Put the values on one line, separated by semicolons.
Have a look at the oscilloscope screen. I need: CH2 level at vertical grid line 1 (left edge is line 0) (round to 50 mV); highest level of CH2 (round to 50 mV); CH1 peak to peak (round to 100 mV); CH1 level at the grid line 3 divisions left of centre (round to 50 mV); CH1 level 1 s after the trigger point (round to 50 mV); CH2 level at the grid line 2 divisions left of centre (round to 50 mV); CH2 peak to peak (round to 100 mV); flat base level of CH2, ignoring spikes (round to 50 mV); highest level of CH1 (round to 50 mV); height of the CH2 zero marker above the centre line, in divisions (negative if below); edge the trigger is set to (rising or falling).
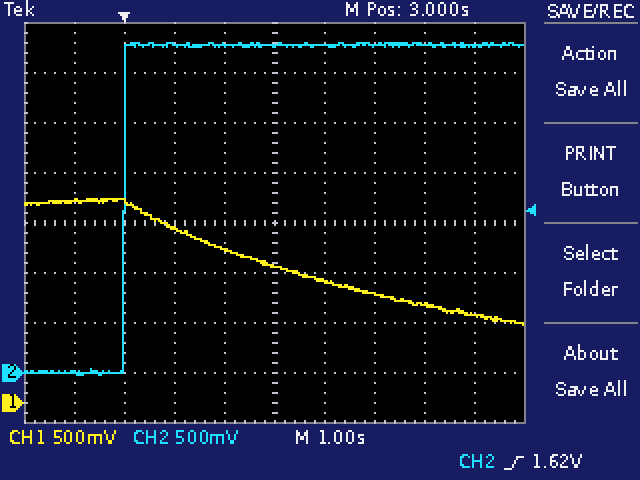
0 mV; 3.30 V; 1.30 V; 2.00 V; 1.75 V; 3.30 V; 3.30 V; 0 mV; 2.05 V; -3.0 div; rising
